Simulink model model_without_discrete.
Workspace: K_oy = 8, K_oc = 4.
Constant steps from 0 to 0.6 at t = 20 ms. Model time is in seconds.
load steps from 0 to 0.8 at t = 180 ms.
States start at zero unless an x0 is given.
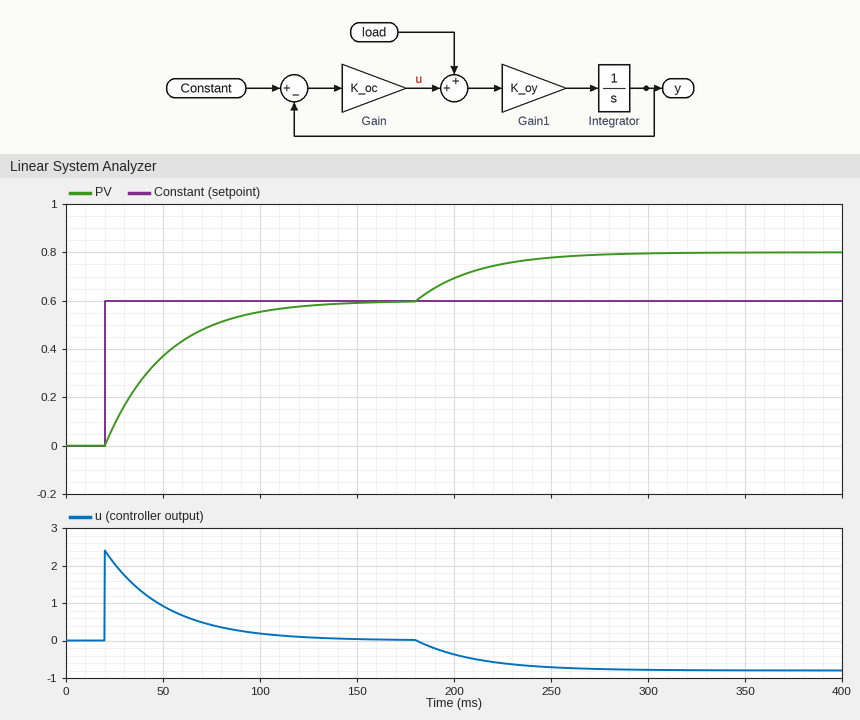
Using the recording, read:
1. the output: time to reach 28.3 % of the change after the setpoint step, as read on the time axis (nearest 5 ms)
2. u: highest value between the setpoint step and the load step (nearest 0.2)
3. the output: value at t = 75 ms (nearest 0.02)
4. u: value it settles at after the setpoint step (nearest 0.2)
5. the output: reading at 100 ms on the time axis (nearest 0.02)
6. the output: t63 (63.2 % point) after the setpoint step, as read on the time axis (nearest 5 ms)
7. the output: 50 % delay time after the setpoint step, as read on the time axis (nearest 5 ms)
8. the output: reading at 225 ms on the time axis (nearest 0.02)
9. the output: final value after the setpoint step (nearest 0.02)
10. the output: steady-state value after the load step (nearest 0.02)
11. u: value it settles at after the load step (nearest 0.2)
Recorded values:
30 ms
2.4
0.50
0.0
0.56
50 ms
40 ms
0.76
0.60
0.80
-0.8
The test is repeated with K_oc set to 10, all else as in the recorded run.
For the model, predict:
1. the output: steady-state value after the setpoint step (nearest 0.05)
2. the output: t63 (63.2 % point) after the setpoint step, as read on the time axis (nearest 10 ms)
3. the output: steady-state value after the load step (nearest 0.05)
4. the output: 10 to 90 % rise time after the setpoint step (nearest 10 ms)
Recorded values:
0.60
30 ms
0.70
30 ms
